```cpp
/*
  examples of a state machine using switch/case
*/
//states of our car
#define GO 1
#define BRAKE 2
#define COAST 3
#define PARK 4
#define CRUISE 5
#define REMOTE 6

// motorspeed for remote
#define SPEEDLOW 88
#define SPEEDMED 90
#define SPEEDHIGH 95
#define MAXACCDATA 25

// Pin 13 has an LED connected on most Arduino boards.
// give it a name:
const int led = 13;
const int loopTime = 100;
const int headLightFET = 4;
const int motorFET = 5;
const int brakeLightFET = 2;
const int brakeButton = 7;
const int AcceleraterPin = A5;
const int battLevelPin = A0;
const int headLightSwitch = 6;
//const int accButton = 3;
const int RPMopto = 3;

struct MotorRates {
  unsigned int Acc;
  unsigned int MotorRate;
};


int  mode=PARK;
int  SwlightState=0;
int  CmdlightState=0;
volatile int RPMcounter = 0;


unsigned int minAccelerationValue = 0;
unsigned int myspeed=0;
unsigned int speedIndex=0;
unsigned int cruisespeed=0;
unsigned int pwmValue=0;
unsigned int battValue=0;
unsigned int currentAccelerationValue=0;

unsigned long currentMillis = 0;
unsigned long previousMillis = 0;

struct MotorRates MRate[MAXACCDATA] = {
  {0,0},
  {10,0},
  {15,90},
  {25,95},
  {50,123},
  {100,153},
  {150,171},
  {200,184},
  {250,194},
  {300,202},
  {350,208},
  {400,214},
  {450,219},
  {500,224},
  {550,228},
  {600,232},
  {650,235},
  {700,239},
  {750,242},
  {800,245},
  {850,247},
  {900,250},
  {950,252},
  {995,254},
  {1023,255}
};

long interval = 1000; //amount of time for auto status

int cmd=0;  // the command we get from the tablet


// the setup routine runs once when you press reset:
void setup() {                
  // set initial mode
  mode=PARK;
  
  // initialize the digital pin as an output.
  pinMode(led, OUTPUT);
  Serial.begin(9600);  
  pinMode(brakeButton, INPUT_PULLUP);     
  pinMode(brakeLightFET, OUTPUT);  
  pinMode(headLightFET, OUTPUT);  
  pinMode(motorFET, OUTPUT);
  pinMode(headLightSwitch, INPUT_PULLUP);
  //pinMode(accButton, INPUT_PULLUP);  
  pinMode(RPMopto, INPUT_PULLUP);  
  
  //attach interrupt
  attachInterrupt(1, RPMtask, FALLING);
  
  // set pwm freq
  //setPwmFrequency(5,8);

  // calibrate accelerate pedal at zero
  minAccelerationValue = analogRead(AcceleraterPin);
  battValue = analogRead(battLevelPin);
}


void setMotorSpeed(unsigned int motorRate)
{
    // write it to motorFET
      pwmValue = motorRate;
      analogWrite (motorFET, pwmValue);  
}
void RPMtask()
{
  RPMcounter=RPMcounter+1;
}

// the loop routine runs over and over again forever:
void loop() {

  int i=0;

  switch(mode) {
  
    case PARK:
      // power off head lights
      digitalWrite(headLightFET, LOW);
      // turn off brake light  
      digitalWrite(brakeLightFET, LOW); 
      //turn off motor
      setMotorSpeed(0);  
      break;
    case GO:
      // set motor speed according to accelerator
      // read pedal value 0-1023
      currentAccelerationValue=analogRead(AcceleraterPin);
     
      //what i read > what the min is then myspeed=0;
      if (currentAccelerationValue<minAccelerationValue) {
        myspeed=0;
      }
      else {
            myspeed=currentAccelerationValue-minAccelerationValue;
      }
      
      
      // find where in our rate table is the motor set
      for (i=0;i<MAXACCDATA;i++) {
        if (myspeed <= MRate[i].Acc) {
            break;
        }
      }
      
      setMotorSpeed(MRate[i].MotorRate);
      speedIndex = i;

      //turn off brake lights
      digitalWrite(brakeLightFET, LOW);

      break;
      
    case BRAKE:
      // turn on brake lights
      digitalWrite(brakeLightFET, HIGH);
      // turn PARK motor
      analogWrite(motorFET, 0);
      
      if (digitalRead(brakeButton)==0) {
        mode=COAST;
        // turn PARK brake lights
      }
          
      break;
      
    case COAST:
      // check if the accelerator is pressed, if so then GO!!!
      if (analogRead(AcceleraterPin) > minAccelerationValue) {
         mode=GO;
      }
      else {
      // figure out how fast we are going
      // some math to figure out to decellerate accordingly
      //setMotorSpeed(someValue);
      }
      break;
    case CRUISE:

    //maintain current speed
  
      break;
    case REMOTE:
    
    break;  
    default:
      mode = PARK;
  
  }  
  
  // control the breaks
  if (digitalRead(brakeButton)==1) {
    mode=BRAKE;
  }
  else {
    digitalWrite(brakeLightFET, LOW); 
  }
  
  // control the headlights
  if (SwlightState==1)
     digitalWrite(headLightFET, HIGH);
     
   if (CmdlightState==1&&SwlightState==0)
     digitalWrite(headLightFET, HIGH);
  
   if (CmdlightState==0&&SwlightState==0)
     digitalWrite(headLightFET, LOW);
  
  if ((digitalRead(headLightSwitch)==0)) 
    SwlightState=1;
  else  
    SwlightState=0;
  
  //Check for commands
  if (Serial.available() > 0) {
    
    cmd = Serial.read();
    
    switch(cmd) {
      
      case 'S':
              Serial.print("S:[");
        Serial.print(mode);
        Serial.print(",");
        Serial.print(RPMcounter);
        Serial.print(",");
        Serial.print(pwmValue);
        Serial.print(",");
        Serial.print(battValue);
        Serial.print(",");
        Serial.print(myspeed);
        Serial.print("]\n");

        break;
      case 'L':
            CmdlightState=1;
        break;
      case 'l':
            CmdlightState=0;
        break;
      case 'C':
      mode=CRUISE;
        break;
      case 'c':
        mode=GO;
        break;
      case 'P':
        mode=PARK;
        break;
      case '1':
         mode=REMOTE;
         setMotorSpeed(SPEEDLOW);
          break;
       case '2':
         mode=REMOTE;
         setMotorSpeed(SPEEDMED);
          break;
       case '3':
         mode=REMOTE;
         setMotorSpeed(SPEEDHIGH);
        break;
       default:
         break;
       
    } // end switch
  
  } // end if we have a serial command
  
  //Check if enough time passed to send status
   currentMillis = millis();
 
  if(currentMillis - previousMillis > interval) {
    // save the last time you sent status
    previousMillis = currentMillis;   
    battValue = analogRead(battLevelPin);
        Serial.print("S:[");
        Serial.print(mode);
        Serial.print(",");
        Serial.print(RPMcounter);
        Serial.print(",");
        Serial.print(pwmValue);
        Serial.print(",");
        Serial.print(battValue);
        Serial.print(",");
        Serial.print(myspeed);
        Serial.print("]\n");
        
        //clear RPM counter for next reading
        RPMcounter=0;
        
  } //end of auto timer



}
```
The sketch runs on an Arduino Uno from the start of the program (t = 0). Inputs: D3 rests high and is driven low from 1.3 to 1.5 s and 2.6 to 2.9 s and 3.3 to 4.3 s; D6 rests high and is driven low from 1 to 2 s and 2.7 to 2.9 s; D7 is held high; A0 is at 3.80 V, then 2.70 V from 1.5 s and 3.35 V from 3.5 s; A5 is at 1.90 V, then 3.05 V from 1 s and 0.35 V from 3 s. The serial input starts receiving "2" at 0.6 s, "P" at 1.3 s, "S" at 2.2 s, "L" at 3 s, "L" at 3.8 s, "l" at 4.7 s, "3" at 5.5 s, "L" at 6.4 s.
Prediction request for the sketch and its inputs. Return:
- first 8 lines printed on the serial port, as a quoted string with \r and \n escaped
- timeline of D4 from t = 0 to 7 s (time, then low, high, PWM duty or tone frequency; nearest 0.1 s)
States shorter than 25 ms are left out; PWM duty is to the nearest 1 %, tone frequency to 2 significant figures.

"S:[2,0,90,778,0]\nS:[2,1,0,552,0]\nS:[2,0,0,552,0]\nS:[2,1,0,552,0]\nS:[2,1,0,686,0]\nS:[2,0,0,686,0]\nS:[2,0,95,686,0]\nS:[2,0,95,686,0]\n"
0 s low; 1 s high; 2 s low; 2.7 s high; 2.9 s low; 3 s high; 4.7 s low; 6.4 s high
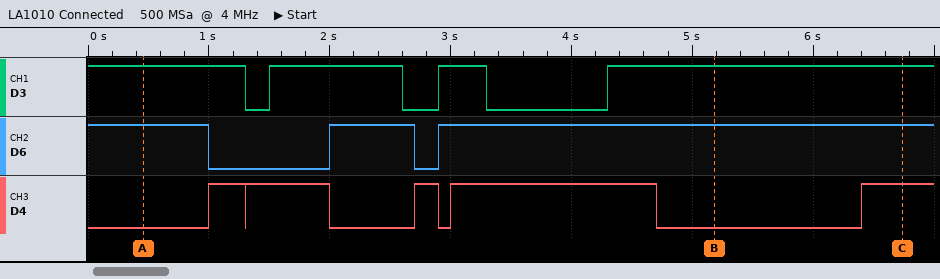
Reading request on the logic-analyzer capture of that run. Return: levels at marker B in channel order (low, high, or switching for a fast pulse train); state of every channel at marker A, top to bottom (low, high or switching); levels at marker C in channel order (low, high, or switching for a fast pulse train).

D3 high, D6 high, D4 low
D3 high, D6 high, D4 low
D3 high, D6 high, D4 high
